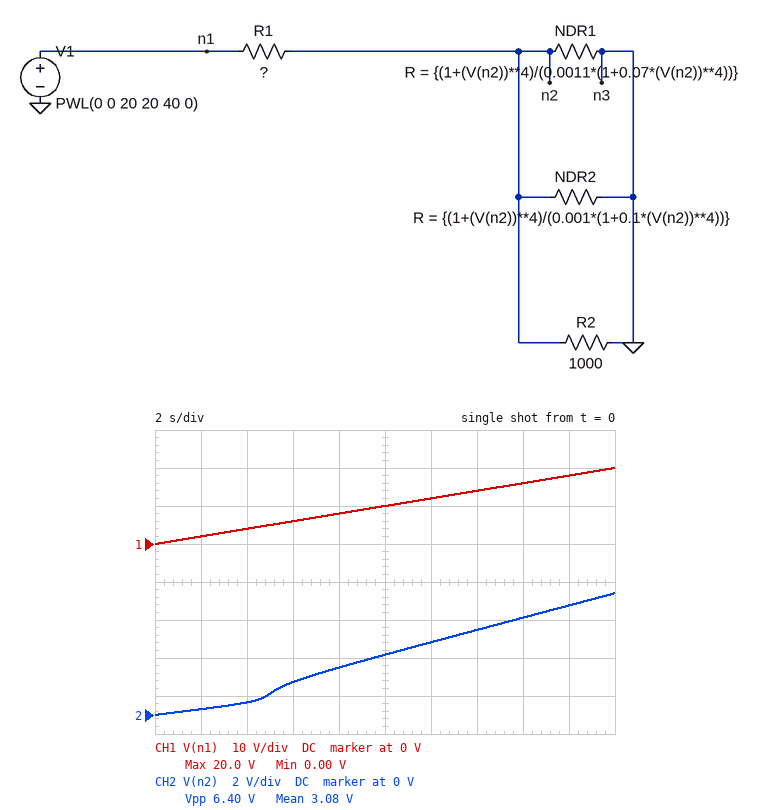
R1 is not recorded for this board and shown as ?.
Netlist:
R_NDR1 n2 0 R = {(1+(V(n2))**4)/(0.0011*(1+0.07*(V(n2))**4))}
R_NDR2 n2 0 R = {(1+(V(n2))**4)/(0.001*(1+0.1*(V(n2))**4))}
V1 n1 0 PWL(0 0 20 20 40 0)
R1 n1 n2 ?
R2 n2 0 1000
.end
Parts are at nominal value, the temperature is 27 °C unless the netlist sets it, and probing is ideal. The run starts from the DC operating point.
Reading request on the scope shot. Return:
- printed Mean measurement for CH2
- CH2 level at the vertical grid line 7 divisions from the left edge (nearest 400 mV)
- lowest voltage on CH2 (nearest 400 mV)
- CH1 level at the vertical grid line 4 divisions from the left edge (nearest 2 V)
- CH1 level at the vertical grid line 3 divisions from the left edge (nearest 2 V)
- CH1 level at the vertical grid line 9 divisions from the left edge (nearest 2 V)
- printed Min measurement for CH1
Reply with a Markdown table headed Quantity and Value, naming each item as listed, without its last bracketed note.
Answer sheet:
| Quantity | Value |
|---|---|
| printed Mean measurement for CH2 | 3.08 V |
| CH2 level at the vertical grid line 7 divisions from the left edge | 4.4 V |
| lowest voltage on CH2 | 0 V |
| CH1 level at the vertical grid line 4 divisions from the left edge | 8 V |
| CH1 level at the vertical grid line 3 divisions from the left edge | 6 V |
| CH1 level at the vertical grid line 9 divisions from the left edge | 18 V |
| printed Min measurement for CH1 | 0.00 V |
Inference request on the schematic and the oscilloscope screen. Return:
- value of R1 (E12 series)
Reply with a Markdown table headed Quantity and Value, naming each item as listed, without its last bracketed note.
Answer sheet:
| Quantity | Value |
|---|---|
| value of R1 | 1.8 kΩ |
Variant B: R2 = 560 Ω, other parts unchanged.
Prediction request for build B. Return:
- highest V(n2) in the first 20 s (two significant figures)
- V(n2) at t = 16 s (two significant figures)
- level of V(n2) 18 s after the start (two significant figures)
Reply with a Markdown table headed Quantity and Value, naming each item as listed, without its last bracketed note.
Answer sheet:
| Quantity | Value |
|---|---|
| highest V(n2) in the first 20 s | 4.4 V |
| V(n2) at t = 16 s | 3.5 V |
| level of V(n2) 18 s after the start | 4.0 V |
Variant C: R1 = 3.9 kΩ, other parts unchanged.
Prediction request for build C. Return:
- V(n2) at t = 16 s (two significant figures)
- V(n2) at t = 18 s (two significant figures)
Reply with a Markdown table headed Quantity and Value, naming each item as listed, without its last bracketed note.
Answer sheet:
| Quantity | Value |
|---|---|
| V(n2) at t = 16 s | 2.8 V |
| V(n2) at t = 18 s | 3.2 V |
